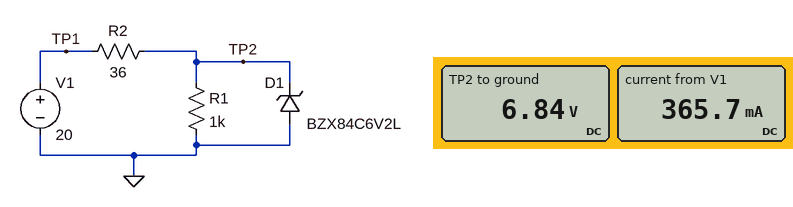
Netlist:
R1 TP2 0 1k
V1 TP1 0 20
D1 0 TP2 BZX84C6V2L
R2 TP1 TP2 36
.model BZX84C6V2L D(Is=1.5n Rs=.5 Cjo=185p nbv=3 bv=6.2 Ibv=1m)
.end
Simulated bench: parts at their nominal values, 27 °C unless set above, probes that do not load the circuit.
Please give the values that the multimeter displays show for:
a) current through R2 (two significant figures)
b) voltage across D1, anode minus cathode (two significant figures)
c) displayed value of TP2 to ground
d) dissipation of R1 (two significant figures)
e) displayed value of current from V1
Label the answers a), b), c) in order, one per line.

a) 370 mA
b) -6.8 V
c) 6.84 V
d) 47 mW
e) 365.7 mA
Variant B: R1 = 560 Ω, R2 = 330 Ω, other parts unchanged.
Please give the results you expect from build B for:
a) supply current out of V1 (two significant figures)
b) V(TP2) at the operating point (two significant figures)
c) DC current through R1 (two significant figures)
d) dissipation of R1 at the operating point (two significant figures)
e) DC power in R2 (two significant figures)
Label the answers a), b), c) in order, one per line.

a) 41 mA
b) 6.5 V
c) 12 mA
d) 75 mW
e) 550 mW
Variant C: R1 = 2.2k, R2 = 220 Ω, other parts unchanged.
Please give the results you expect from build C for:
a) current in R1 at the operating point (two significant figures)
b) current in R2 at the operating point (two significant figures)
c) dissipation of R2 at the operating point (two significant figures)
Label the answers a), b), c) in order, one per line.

a) 3.0 mA
b) 61 mA
c) 820 mW
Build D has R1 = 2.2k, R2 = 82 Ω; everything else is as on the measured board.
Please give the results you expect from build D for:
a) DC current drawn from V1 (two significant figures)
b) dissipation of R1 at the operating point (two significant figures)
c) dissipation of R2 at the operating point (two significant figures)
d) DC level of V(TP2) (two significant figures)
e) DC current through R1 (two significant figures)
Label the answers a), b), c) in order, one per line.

a) 160 mA
b) 20 mW
c) 2.2 W
d) 6.7 V
e) 3.0 mA
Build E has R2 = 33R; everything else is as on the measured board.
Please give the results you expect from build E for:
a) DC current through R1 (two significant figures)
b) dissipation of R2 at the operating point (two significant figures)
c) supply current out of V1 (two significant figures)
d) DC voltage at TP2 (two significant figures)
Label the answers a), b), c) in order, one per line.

a) 6.9 mA
b) 5.2 W
c) 400 mA
d) 6.9 V
